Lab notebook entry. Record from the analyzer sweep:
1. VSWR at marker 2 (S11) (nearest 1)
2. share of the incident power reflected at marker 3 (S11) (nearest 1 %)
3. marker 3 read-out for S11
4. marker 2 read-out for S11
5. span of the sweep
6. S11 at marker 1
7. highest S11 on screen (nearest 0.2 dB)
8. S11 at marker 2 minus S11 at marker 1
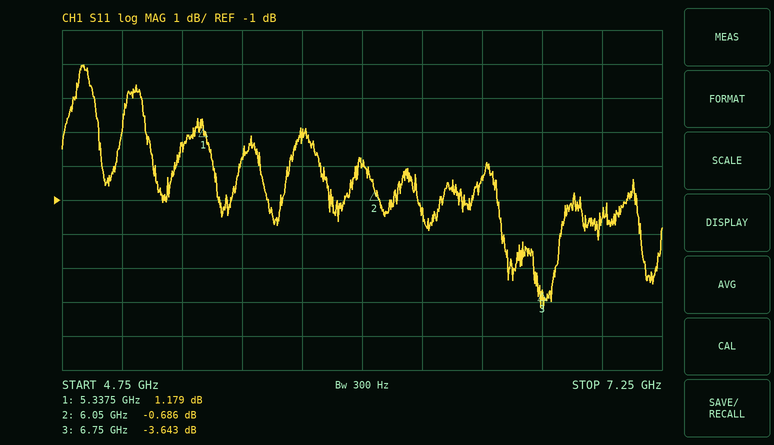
25
43 %
-3.643 dB
-0.686 dB
2.5 GHz
1.179 dB
3.0 dB
-1.865 dB
